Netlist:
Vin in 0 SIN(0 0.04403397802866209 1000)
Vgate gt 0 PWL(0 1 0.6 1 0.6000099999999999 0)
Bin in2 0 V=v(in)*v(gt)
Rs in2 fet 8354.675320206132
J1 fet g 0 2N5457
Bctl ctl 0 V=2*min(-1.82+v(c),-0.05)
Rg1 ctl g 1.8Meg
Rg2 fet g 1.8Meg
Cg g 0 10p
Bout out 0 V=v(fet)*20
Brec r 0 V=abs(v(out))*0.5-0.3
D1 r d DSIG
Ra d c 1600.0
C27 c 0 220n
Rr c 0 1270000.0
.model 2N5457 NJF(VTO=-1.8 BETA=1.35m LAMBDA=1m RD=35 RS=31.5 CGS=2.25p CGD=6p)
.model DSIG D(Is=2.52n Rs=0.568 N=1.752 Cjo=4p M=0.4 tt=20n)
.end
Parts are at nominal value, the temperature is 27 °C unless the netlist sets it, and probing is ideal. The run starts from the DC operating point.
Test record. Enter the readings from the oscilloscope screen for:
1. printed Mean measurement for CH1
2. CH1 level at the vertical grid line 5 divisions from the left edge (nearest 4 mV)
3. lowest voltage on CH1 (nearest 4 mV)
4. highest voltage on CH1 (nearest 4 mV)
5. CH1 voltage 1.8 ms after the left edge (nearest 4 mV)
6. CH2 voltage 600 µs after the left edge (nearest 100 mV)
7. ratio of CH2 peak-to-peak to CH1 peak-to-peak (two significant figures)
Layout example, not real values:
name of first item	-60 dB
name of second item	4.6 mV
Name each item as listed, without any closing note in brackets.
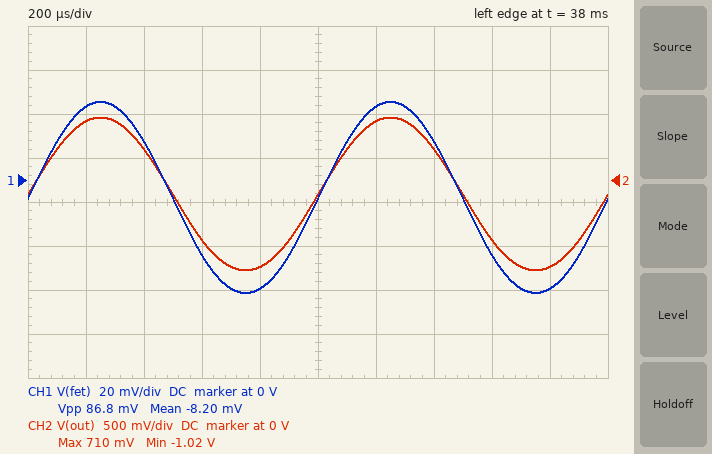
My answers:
printed Mean measurement for CH1	-8.20 mV
CH1 level at the vertical grid line 5 divisions from the left edge	-8 mV
lowest voltage on CH1	-52 mV
highest voltage on CH1	36 mV
CH1 voltage 1.8 ms after the left edge	-48 mV
CH2 voltage 600 µs after the left edge	-700 mV
ratio of CH2 peak-to-peak to CH1 peak-to-peak	20
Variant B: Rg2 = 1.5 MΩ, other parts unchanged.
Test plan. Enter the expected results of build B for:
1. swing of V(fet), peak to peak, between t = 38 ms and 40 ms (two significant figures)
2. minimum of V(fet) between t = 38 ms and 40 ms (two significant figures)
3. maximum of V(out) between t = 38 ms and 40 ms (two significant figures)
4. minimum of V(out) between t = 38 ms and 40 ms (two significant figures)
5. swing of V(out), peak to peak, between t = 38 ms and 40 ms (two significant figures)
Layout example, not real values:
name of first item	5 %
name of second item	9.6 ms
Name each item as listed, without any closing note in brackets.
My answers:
swing of V(fet), peak to peak, between t = 38 ms and 40 ms	21 mV
minimum of V(fet) between t = 38 ms and 40 ms	-13 mV
maximum of V(out) between t = 38 ms and 40 ms	170 mV
minimum of V(out) between t = 38 ms and 40 ms	-260 mV
swing of V(out), peak to peak, between t = 38 ms and 40 ms	430 mV
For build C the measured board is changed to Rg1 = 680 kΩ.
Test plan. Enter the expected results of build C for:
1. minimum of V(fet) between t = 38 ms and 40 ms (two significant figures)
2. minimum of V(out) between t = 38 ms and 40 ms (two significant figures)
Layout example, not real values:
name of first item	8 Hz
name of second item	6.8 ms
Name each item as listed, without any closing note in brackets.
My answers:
minimum of V(fet) between t = 38 ms and 40 ms	-56 mV
minimum of V(out) between t = 38 ms and 40 ms	-1.1 V
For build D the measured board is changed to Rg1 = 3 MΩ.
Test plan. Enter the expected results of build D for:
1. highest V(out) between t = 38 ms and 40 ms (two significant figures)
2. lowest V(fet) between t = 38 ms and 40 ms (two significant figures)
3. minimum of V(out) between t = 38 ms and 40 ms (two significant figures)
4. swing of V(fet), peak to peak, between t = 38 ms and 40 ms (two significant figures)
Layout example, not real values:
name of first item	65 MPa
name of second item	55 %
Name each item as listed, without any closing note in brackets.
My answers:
highest V(out) between t = 38 ms and 40 ms	75 mV
lowest V(fet) between t = 38 ms and 40 ms	-5.0 mV
minimum of V(out) between t = 38 ms and 40 ms	-100 mV
swing of V(fet), peak to peak, between t = 38 ms and 40 ms	8.8 mV
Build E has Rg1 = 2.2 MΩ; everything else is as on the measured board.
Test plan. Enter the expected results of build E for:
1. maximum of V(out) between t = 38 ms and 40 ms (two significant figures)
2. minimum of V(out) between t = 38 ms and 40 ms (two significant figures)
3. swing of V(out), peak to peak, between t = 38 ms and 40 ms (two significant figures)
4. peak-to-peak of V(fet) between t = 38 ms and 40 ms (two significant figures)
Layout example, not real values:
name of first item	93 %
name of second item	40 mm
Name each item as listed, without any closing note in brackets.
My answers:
maximum of V(out) between t = 38 ms and 40 ms	160 mV
minimum of V(out) between t = 38 ms and 40 ms	-230 mV
swing of V(out), peak to peak, between t = 38 ms and 40 ms	390 mV
peak-to-peak of V(fet) between t = 38 ms and 40 ms	20 mV
